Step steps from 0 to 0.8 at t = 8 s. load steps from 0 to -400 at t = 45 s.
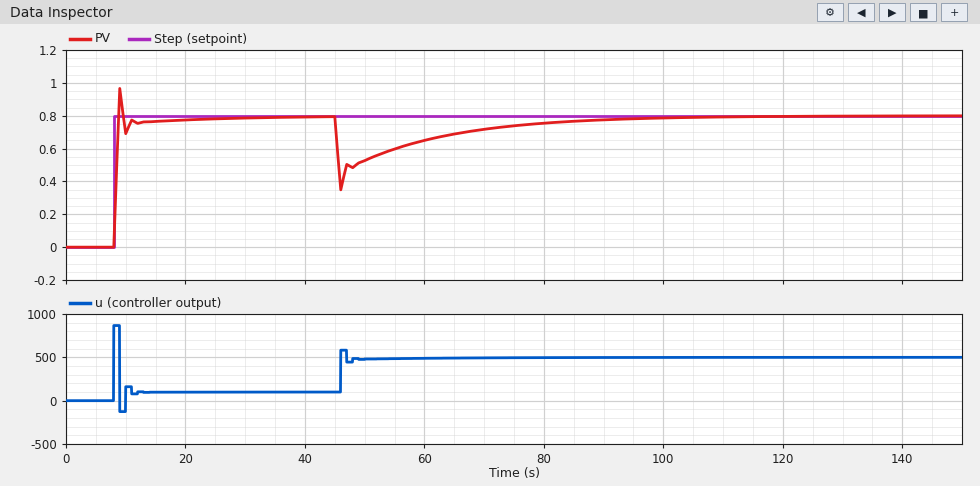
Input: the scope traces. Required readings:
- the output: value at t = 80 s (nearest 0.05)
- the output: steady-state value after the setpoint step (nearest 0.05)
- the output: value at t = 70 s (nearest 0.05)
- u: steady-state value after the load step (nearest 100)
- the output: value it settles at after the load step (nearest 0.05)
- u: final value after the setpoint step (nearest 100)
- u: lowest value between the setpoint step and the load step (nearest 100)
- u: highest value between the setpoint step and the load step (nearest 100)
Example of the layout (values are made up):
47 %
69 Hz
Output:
0.75
0.80
0.70
500
0.80
100
-100
900
